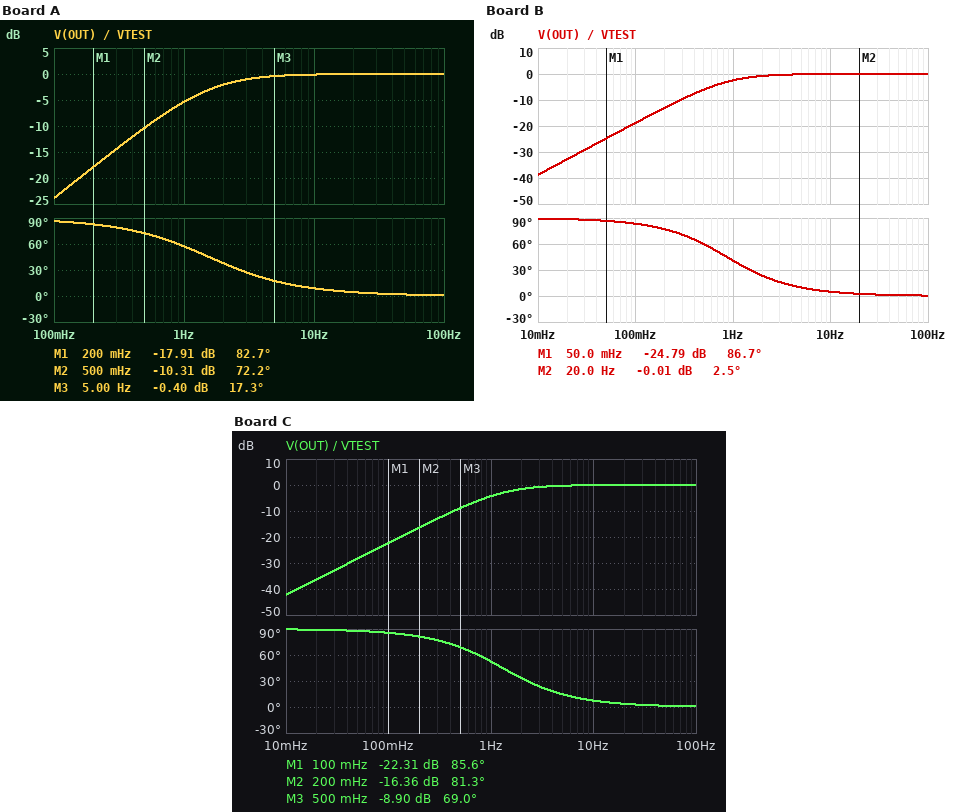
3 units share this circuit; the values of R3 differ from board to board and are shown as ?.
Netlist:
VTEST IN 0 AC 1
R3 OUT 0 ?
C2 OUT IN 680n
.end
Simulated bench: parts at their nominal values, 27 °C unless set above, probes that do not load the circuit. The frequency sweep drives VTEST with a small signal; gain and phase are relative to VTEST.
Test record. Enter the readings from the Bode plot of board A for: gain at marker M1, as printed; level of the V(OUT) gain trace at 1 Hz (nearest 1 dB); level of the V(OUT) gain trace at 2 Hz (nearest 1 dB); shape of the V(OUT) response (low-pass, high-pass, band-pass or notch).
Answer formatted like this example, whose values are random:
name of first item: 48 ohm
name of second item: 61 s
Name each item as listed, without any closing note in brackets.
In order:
gain at marker M1, as printed: -17.91 dB
level of the V(OUT) gain trace at 1 Hz: -5 dB
level of the V(OUT) gain trace at 2 Hz: -2 dB
shape of the V(OUT) response: high-pass
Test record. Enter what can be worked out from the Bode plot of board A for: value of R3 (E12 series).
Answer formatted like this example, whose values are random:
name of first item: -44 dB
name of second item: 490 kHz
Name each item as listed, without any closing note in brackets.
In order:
value of R3: 150 kΩ
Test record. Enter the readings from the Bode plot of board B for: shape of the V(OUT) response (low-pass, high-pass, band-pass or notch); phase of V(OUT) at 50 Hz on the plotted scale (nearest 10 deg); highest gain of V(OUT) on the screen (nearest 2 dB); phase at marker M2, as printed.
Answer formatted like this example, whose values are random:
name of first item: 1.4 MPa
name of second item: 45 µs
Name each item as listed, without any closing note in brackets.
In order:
shape of the V(OUT) response: high-pass
phase of V(OUT) at 50 Hz on the plotted scale: 0 deg
highest gain of V(OUT) on the screen: 0 dB
phase at marker M2, as printed: 2.5 deg
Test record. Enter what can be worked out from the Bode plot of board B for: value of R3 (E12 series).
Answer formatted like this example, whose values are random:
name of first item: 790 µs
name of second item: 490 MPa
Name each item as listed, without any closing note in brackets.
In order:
value of R3: 270 kΩ
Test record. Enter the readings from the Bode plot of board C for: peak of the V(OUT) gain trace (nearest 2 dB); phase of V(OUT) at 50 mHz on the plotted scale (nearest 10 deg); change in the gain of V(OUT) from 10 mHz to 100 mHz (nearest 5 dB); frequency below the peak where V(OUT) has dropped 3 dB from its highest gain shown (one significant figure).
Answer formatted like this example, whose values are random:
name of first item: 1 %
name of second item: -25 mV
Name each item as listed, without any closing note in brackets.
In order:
peak of the V(OUT) gain trace: 0 dB
phase of V(OUT) at 50 mHz on the plotted scale: 90 deg
change in the gain of V(OUT) from 10 mHz to 100 mHz: 20 dB
frequency below the peak where V(OUT) has dropped 3 dB from its highest gain shown: 1 Hz
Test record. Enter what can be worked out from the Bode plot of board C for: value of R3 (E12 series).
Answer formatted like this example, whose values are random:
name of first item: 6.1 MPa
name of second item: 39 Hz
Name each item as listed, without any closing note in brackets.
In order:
value of R3: 180 kΩ
